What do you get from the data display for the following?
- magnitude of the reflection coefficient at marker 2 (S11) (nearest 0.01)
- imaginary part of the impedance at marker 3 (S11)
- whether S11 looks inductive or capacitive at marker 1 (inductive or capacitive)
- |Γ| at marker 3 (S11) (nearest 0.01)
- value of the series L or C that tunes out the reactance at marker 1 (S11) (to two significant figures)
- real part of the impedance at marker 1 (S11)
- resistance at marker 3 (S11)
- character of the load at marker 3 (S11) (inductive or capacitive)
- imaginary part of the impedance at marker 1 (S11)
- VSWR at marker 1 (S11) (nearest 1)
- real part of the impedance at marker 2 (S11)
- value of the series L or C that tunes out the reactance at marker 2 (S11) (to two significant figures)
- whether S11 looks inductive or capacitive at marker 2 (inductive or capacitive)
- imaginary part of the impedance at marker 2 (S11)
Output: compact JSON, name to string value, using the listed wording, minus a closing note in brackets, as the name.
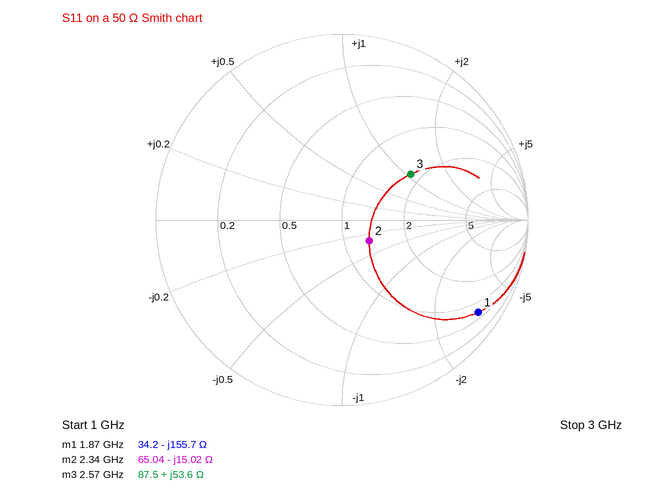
{"magnitude of the reflection coefficient at marker 2 (S11)": "0.18", "imaginary part of the impedance at marker 3": "+53.6 Ω", "whether S11 looks inductive or capacitive at marker 1": "capacitive", "|Γ| at marker 3 (S11)": "0.44", "value of the series L or C that tunes out the reactance at marker 1 (S11)": "13 nH", "real part of the impedance at marker 1": "34.2 Ω", "resistance at marker 3": "87.5 Ω", "character of the load at marker 3 (S11)": "inductive", "imaginary part of the impedance at marker 1": "-155.7 Ω", "VSWR at marker 1 (S11)": "16", "real part of the impedance at marker 2": "65.04 Ω", "value of the series L or C that tunes out the reactance at marker 2 (S11)": "1.0 nH", "whether S11 looks inductive or capacitive at marker 2": "capacitive", "imaginary part of the impedance at marker 2": "-15.02 Ω"}
